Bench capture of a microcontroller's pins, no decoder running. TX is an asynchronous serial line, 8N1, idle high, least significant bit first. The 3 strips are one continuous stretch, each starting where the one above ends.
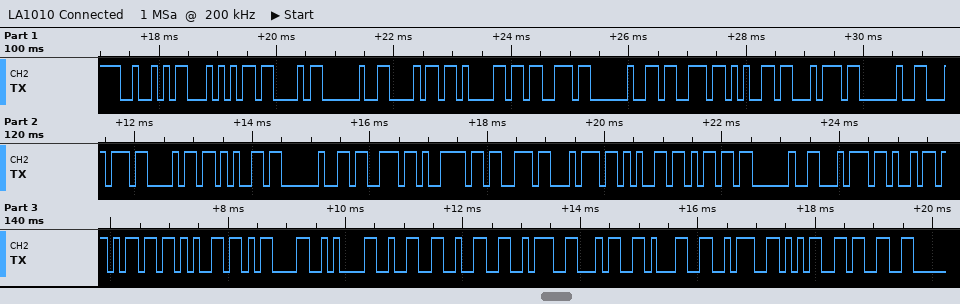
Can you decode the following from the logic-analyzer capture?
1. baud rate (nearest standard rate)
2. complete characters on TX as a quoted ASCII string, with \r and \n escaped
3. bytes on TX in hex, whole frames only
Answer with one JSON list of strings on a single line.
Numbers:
["9600 baud", "\"RTC has set the system time\\r\\n22:41:53\"", "52 54 43 20 68 61 73 20 73 65 74 20 74 68 65 20 73 79 73 74 65 6D 20 74 69 6D 65 0D 0A 32 32 3A 34 31 3A 35 33"]
